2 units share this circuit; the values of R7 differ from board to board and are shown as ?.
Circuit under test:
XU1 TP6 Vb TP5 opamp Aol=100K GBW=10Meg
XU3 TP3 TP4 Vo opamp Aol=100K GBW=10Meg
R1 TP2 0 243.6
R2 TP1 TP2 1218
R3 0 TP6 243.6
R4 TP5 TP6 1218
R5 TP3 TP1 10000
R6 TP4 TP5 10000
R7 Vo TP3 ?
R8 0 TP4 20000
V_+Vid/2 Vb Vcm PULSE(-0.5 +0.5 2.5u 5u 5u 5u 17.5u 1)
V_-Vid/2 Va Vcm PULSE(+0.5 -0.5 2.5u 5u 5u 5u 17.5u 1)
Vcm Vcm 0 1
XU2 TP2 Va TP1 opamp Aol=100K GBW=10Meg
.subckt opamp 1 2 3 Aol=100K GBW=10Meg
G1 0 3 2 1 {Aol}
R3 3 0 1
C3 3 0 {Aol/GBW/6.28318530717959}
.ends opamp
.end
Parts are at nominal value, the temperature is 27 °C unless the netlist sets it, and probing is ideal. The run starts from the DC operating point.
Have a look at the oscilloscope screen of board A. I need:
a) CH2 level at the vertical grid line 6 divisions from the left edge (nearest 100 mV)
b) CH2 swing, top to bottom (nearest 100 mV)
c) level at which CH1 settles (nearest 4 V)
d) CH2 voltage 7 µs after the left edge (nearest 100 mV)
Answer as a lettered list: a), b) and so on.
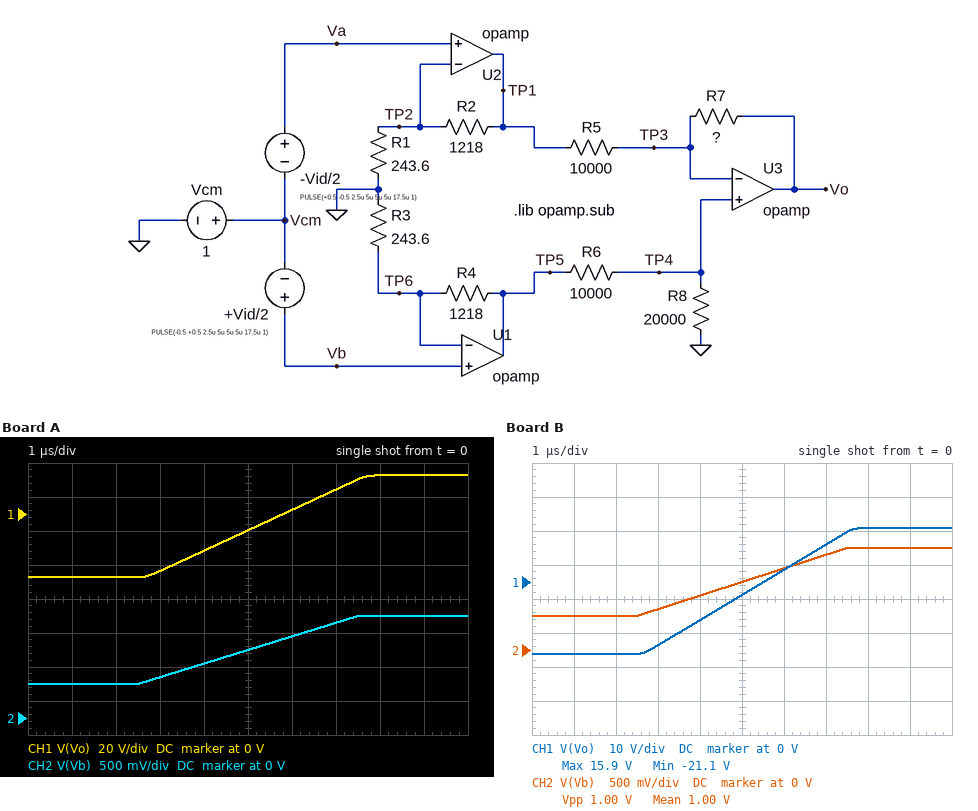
a) 1.2 V
b) 1.0 V
c) 24 V
d) 1.4 V
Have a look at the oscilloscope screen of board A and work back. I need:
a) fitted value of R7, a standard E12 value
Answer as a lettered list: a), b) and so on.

a) 56 kΩ
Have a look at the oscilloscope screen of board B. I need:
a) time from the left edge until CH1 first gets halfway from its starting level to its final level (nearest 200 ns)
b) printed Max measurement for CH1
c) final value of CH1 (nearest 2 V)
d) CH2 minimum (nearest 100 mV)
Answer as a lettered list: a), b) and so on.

a) 5.2 µs
b) 15.9 V
c) 16 V
d) 500 mV
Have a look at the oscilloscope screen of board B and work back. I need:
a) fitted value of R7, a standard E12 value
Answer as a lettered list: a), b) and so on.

a) 33 kΩ
